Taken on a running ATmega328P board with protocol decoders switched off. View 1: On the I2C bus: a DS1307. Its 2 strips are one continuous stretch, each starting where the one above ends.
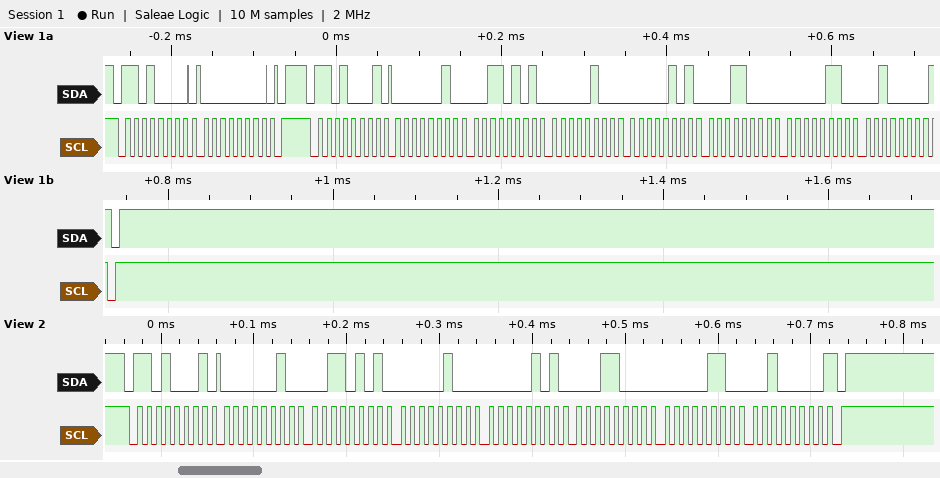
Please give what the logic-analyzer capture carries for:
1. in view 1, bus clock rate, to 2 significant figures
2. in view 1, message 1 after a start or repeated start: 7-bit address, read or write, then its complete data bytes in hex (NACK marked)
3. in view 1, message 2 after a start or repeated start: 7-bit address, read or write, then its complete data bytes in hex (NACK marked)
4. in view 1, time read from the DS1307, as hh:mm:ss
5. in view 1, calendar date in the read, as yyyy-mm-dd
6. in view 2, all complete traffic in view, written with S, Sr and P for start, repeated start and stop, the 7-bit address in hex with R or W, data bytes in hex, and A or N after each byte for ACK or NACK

100 kHz
0x68 write: 00
0x68 read: 02 35 04 05 18 06 20 NACK
04:35:02
2020-06-18
S 68R A 02 A 35 A 04 A 05 A 18 A 06 A 20 N P
